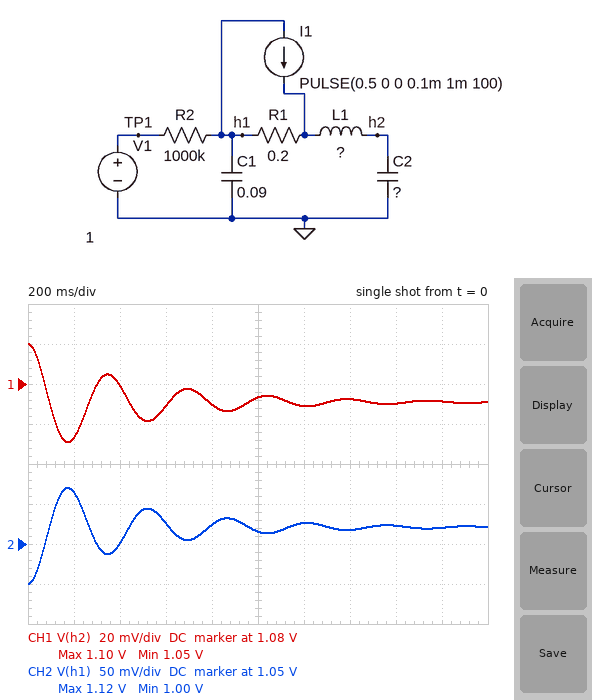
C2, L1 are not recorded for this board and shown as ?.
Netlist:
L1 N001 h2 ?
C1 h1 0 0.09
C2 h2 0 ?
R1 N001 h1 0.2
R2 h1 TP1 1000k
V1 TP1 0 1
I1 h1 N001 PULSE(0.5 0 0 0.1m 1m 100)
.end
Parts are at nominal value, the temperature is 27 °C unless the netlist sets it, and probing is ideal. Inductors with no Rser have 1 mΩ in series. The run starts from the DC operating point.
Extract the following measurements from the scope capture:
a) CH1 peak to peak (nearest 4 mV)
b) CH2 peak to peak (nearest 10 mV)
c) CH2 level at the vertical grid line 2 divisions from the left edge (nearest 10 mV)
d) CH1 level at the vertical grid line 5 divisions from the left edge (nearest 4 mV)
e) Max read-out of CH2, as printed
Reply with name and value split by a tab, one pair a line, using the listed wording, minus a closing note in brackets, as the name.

CH1 peak to peak	48 mV
CH2 peak to peak	120 mV
CH2 level at the vertical grid line 2 divisions from the left edge	1.05 V
CH1 level at the vertical grid line 5 divisions from the left edge	1.072 V
Max read-out of CH2, as printed	1.12 V
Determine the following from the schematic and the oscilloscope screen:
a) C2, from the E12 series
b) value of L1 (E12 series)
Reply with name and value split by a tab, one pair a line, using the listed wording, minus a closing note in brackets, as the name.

C2, from the E12 series	220 mF
value of L1	47 mH
